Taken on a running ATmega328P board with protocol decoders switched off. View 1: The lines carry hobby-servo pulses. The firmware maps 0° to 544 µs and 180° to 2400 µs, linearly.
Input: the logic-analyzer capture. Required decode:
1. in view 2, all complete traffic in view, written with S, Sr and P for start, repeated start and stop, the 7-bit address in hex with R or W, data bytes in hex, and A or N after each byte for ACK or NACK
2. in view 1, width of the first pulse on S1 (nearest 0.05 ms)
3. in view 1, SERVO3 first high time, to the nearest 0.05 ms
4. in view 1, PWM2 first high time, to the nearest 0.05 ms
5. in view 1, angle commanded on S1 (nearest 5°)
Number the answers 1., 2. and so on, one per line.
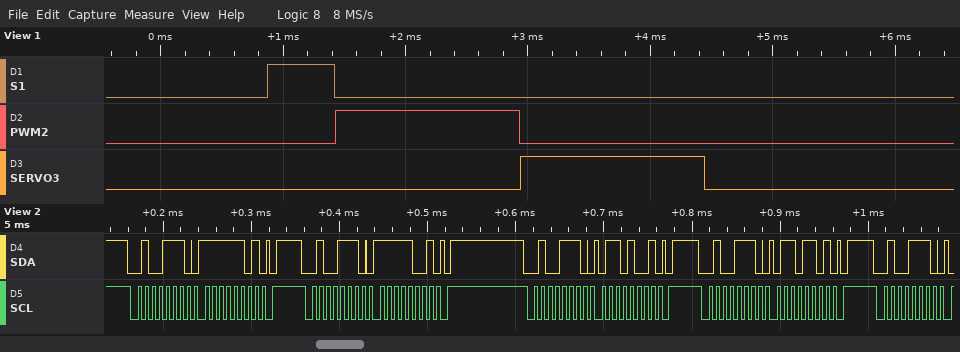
1. S 27W A FD A P S 27W A F9 A P S 27W A 69 A P S 27W A 6D A P S 27W A
2. 0.55 ms
3. 1.50 ms
4. 1.50 ms
5. 0°
